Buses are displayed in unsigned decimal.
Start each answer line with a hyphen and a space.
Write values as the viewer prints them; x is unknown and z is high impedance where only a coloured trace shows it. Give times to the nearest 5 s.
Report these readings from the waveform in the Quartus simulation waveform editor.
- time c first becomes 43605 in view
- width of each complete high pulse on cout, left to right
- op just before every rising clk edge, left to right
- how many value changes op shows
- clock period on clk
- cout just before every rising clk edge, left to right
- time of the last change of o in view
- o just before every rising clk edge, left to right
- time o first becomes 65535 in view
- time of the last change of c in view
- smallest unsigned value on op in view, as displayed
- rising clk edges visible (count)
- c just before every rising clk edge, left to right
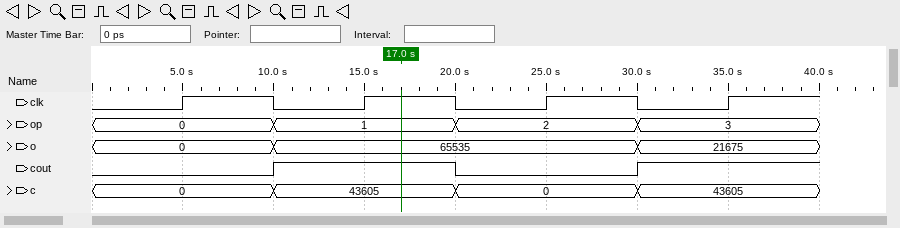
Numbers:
- 10 s
- 10 s
- 0, 1, 2, 3
- 3
- 10 s
- 0 1 0 1
- 30 s
- 0, 65535, 65535, 21675
- 10 s
- 30 s
- 0
- 4
- 0, 43605, 0, 43605
